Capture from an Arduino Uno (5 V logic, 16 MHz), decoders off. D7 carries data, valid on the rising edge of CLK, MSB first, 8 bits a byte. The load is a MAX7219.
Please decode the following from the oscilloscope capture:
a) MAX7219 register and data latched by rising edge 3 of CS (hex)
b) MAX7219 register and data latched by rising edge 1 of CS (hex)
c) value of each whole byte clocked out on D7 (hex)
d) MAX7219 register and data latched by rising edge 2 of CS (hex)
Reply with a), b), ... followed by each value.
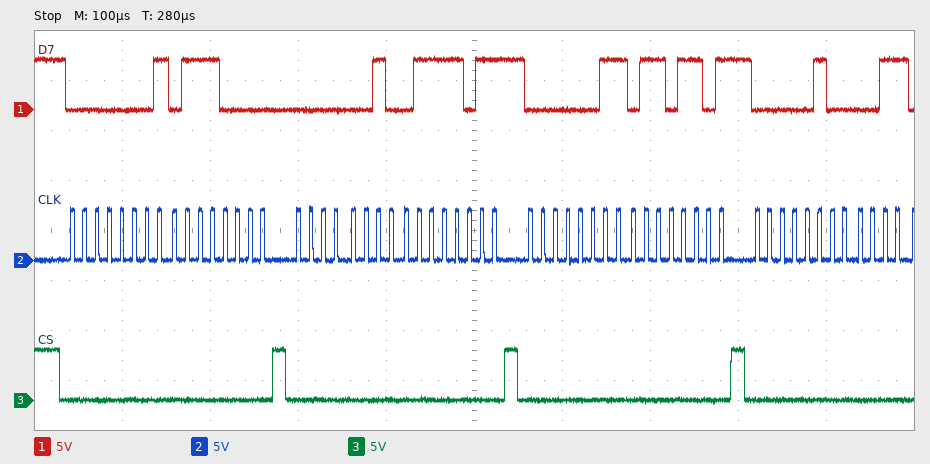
a) register 0x3, data 0x6D
b) register 0x1, data 0x70
c) 01 70 02 7B 03 6D 04
d) register 0x2, data 0x7B
